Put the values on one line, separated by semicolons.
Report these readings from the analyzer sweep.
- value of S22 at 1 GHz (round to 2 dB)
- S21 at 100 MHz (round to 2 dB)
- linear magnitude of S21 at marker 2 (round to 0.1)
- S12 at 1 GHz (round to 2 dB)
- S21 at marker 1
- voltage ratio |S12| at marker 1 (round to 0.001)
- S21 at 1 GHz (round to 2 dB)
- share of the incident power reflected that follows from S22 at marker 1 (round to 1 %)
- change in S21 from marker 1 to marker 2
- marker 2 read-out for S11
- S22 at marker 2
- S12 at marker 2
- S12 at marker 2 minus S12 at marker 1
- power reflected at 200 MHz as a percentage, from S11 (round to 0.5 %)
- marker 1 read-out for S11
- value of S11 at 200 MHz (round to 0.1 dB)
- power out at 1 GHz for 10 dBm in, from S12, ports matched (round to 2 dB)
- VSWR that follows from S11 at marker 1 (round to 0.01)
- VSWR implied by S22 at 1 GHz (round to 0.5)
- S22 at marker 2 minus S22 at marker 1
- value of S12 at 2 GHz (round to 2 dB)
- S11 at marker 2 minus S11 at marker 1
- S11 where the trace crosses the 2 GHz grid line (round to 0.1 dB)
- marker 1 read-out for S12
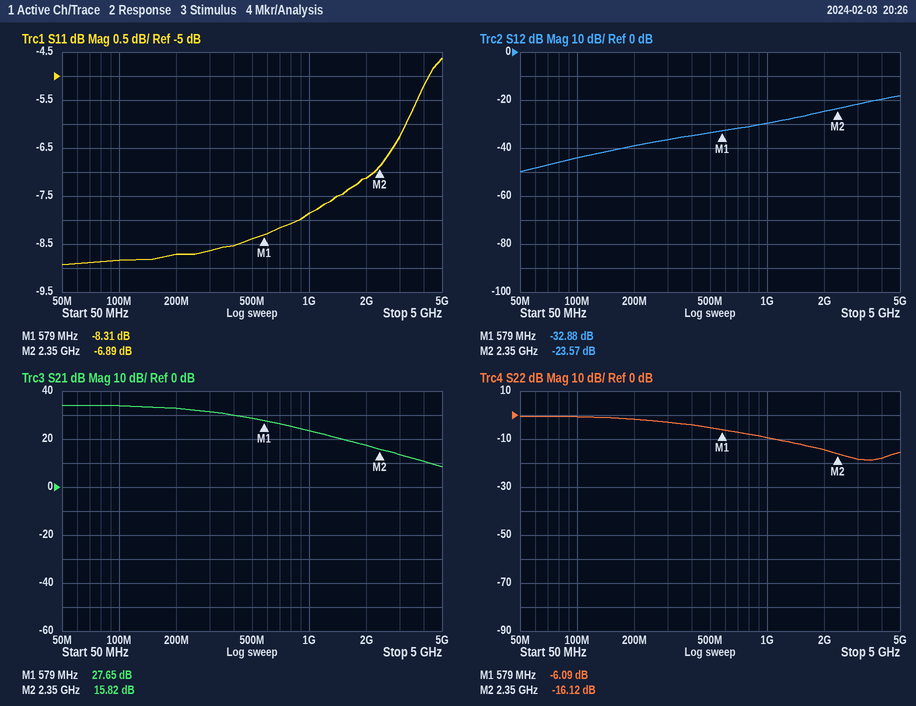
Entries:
-10 dB; 34 dB; 6.2; -30 dB; 27.65 dB; 0.023; 24 dB; 25 %; -11.83 dB; -6.89 dB; -16.12 dB; -23.57 dB; 9.31 dB; 13.5 %; -8.31 dB; -8.7 dB; -20 dBm; 2.25; 2.0; -10.03 dB; -24 dB; 1.42 dB; -7.1 dB; -32.88 dB
